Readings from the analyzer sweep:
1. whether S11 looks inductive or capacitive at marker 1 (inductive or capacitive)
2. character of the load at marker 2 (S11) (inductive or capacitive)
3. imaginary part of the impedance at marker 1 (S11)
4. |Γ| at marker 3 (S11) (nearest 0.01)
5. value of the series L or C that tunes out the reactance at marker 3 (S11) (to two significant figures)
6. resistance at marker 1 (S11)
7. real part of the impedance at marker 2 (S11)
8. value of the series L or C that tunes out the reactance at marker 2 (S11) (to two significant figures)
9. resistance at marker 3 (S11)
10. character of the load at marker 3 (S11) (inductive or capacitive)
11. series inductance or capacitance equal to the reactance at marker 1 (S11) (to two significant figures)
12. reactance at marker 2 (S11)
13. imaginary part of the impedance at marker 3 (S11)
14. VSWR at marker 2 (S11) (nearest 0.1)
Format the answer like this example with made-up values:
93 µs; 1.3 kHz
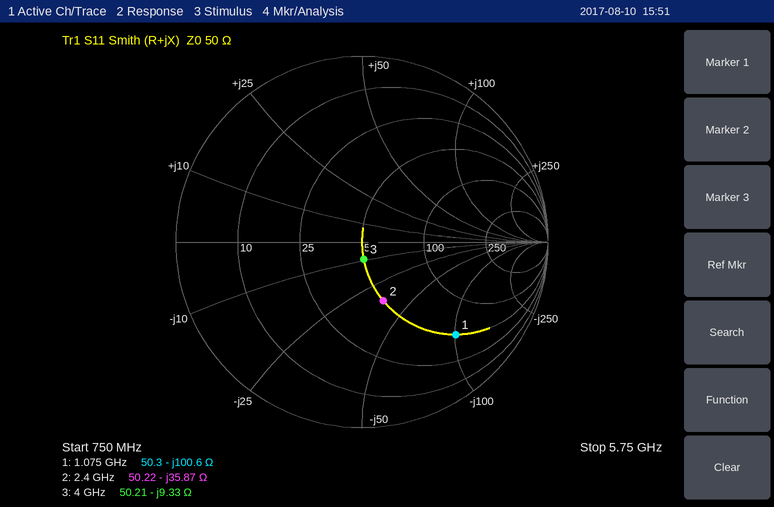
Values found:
capacitive; capacitive; -100.6 Ω; 0.09; 370 pH; 50.3 Ω; 50.22 Ω; 2.4 nH; 50.21 Ω; capacitive; 1.5 pF; -35.87 Ω; -9.33 Ω; 2.0
